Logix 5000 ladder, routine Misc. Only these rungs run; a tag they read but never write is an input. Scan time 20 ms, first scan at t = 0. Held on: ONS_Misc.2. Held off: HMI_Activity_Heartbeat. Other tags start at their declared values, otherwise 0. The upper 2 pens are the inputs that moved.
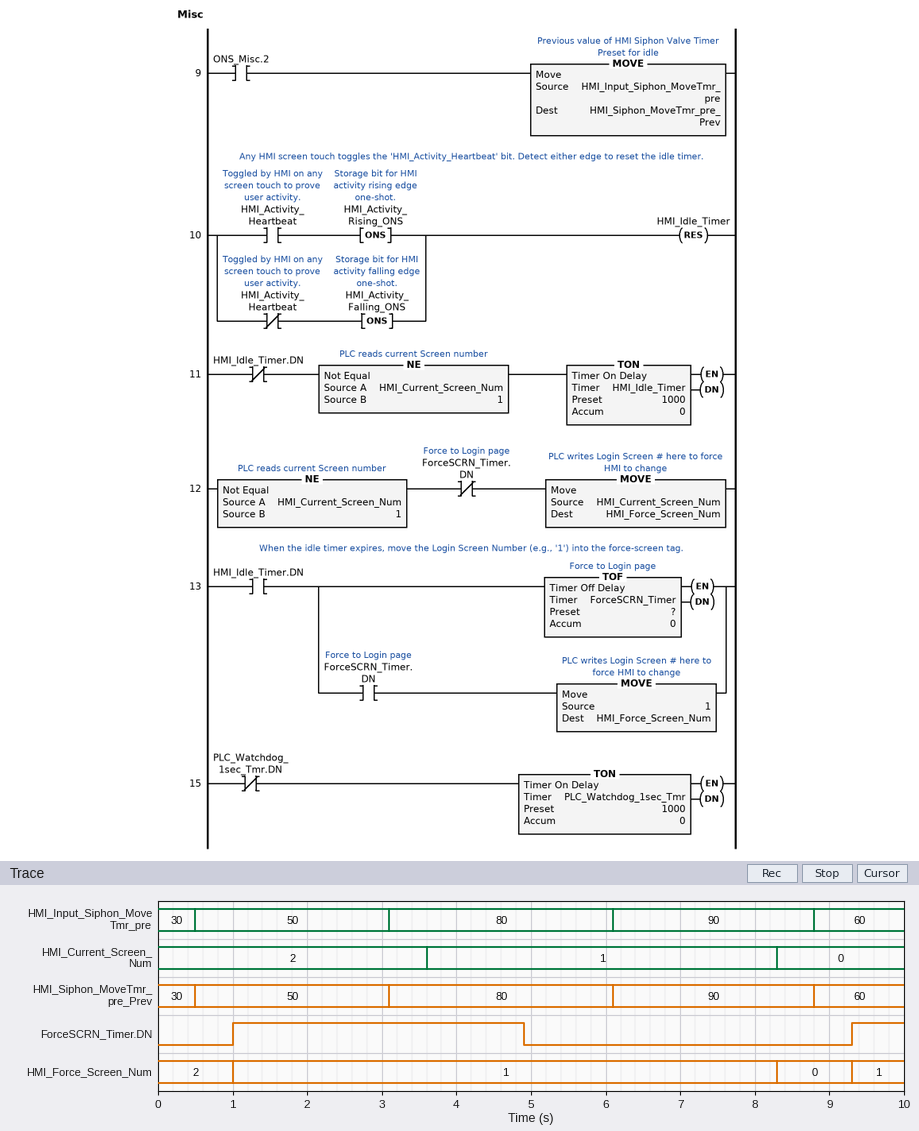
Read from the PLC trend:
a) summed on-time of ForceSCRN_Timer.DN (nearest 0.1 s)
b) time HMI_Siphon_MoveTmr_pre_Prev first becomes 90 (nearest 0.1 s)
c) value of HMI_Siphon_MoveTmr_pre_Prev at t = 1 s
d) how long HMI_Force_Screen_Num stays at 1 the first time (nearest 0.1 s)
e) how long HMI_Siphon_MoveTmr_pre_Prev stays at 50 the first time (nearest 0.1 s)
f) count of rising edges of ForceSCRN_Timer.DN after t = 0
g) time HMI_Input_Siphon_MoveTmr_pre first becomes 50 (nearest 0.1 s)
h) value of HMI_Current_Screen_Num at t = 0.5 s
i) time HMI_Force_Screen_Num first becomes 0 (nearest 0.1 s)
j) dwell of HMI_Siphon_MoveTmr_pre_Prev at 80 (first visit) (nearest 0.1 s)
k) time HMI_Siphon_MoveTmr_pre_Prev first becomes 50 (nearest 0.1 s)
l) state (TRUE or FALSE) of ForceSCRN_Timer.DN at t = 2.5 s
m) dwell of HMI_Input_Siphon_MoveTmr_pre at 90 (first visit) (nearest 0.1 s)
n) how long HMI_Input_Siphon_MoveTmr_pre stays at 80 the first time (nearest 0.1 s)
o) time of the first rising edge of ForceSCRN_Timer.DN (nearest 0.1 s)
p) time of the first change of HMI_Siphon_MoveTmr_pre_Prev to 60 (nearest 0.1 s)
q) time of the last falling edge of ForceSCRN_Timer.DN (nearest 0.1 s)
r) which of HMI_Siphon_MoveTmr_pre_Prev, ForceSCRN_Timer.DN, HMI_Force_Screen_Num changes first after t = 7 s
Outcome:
4.6 s
6.1 s
50
7.3 s
2.6 s
2
0.5 s
2
8.3 s
3.0 s
0.5 s
TRUE
2.7 s
3.0 s
1.0 s
8.8 s
4.9 s
HMI_Force_Screen_Num
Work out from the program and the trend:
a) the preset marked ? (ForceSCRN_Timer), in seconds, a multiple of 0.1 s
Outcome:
1.8 s
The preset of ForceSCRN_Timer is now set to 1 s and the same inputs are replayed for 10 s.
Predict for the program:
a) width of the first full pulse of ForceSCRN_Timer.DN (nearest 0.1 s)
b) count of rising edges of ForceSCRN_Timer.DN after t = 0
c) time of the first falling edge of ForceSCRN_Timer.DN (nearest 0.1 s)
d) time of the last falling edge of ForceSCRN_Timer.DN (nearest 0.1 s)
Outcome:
1.0 s
4
2.0 s
4.1 s
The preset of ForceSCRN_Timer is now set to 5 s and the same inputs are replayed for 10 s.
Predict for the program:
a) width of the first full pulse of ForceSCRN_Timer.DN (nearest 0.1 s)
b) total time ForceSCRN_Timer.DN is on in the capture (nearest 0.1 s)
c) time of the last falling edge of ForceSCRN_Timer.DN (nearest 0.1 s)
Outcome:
7.1 s
7.8 s
8.1 s
